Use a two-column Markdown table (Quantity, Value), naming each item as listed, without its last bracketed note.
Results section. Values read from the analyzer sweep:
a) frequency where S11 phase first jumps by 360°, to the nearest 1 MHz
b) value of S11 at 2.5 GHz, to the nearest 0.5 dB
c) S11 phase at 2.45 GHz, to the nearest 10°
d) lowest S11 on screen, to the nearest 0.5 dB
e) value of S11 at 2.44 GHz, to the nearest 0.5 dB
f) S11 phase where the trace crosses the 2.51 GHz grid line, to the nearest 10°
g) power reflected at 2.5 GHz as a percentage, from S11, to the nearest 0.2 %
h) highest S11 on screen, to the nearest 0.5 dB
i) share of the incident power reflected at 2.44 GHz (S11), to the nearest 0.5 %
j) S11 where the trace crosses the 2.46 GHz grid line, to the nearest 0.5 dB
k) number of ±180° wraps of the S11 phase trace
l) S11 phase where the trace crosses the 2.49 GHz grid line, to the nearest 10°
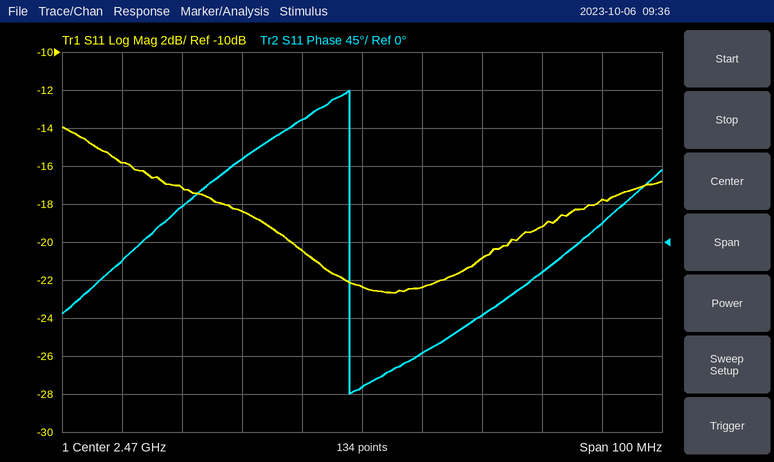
| Quantity | Value |
|---|---|
| frequency where S11 phase first jumps by 360°, to the nearest 1 MHz | 2.468 GHz |
| value of S11 at 2.5 GHz, to the nearest 0.5 dB | -19.0 dB |
| S11 phase at 2.45 GHz, to the nearest 10° | 100° |
| lowest S11 on screen, to the nearest 0.5 dB | -22.5 dB |
| value of S11 at 2.44 GHz, to the nearest 0.5 dB | -17.0 dB |
| S11 phase where the trace crosses the 2.51 GHz grid line, to the nearest 10° | 20° |
| power reflected at 2.5 GHz as a percentage, from S11, to the nearest 0.2 % | 1.2 % |
| highest S11 on screen, to the nearest 0.5 dB | -14.0 dB |
| share of the incident power reflected at 2.44 GHz (S11), to the nearest 0.5 % | 2.0 % |
| S11 where the trace crosses the 2.46 GHz grid line, to the nearest 0.5 dB | -20.5 dB |
| number of ±180° wraps of the S11 phase trace | 1 |
| S11 phase where the trace crosses the 2.49 GHz grid line, to the nearest 10° | -90° |
